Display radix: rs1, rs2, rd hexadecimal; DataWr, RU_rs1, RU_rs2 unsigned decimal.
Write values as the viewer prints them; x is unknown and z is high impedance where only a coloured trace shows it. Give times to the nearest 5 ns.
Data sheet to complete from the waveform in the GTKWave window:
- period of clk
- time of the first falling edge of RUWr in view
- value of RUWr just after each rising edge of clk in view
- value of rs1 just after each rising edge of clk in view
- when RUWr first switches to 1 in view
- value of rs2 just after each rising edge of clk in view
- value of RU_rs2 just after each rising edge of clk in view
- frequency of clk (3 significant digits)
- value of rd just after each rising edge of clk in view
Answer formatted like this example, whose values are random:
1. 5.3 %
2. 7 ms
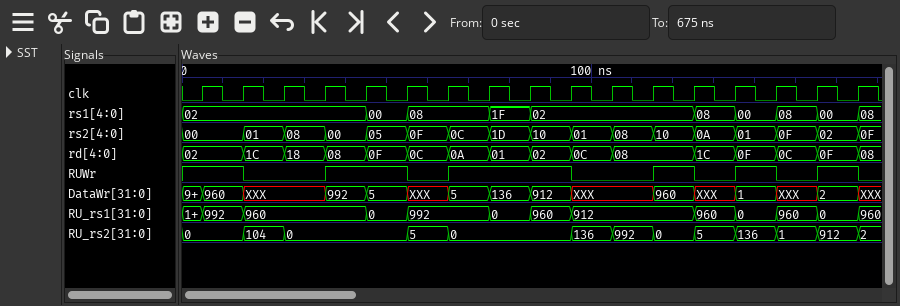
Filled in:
1. 10 ns
2. 15 ns
3. 1 0 0 1 1 0 1 1 1 0 0 1 0 1 0 1 0
4. 02, 02, 02, 02, 00, 08, 08, 1F, 02, 02, 02, 02, 08, 00, 08, 00, 08
5. 35 ns
6. 00, 01, 08, 00, 05, 0F, 0C, 1D, 10, 01, 08, 10, 0A, 01, 0F, 02, 0F
7. 0, 104, 0, 0, 0, 5, 0, 0, 0, 136, 992, 0, 5, 136, 1, 912, 2
8. 100 MHz
9. 02, 1C, 18, 08, 0F, 0C, 0A, 01, 02, 0C, 08, 08, 1C, 0F, 0C, 0F, 08
